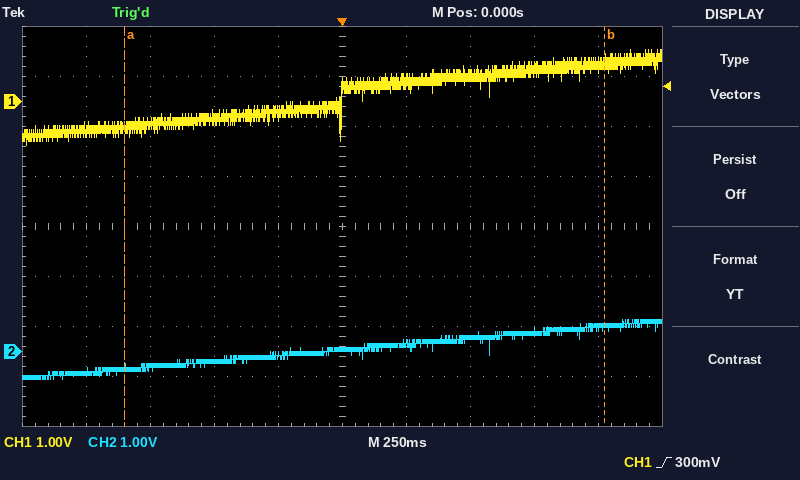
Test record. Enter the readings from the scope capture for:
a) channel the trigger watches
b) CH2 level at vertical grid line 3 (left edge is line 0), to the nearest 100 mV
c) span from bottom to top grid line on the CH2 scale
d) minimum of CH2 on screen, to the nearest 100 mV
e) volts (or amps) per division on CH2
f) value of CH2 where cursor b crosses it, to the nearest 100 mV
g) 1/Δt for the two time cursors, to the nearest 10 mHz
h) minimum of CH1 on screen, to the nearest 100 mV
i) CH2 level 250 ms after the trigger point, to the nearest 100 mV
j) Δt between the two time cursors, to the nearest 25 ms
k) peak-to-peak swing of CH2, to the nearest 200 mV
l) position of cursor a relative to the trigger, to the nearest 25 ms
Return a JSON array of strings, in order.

["CH1", "-200 mV", "8 V", "-600 mV", "1 V", "500 mV", "530 mHz", "-900 mV", "200 mV", "1.875 s", "1.2 V", "-850 ms"]
